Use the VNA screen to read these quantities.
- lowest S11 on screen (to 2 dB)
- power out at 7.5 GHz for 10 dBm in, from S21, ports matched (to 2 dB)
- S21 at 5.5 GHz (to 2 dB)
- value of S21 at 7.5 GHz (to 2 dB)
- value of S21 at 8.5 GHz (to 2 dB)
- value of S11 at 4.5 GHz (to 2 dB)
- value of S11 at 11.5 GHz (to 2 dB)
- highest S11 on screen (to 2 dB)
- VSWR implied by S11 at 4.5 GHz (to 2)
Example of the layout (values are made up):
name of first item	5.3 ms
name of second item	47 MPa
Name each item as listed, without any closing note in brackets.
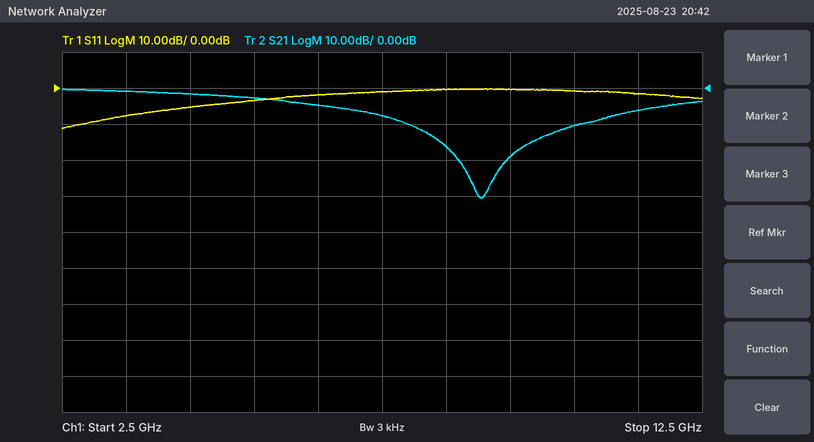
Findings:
lowest S11 on screen	-12 dB
power out at 7.5 GHz for 10 dBm in, from S21, ports matched	2 dBm
S21 at 5.5 GHz	-2 dB
value of S21 at 7.5 GHz	-8 dB
value of S21 at 8.5 GHz	-16 dB
value of S11 at 4.5 GHz	-6 dB
value of S11 at 11.5 GHz	-2 dB
highest S11 on screen	0 dB
VSWR implied by S11 at 4.5 GHz	4
